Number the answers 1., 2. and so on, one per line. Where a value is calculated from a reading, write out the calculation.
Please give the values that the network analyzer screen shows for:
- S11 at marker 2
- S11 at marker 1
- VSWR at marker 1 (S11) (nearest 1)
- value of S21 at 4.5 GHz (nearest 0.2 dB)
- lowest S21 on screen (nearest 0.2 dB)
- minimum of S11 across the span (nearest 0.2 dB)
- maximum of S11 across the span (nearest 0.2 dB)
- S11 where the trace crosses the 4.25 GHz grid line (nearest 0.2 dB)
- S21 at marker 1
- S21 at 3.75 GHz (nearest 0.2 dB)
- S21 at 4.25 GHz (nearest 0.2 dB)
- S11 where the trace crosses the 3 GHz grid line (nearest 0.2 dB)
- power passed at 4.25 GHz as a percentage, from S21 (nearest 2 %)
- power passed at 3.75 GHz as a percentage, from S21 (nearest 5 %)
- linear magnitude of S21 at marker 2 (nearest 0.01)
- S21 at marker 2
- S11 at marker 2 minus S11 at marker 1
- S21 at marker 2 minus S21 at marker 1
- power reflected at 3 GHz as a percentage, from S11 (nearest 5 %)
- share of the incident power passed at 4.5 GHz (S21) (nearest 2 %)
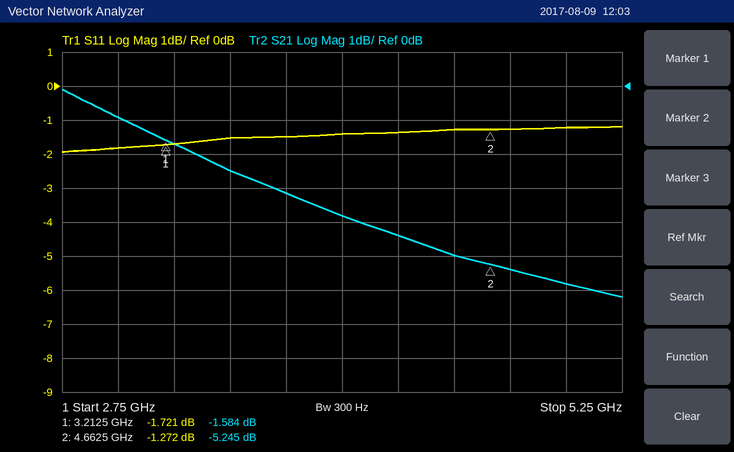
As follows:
1. -1.272 dB
2. -1.721 dB
3. (1 + 0.8203)/(1 − 0.8203) ≈ 10
4. -5.0 dB
5. -6.2 dB
6. -2.0 dB
7. -1.2 dB
8. -1.4 dB
9. -1.584 dB
10. -3.2 dB
11. -4.4 dB
12. -1.8 dB
13. 10^(-4.4/10) ≈ 36 %
14. 10^(-3.2/10) ≈ 47.9 %, so 50 % to the nearest 5 %
15. 10^(-5.245/20) ≈ 0.55
16. -5.245 dB
17. -1.272 − (-1.721) = 0.449 dB
18. -5.245 − (-1.584) = -3.661 dB
19. 10^(-1.8/10) ≈ 66.1 %, so 65 % to the nearest 5 %
20. 10^(-5/10) ≈ 32 %
